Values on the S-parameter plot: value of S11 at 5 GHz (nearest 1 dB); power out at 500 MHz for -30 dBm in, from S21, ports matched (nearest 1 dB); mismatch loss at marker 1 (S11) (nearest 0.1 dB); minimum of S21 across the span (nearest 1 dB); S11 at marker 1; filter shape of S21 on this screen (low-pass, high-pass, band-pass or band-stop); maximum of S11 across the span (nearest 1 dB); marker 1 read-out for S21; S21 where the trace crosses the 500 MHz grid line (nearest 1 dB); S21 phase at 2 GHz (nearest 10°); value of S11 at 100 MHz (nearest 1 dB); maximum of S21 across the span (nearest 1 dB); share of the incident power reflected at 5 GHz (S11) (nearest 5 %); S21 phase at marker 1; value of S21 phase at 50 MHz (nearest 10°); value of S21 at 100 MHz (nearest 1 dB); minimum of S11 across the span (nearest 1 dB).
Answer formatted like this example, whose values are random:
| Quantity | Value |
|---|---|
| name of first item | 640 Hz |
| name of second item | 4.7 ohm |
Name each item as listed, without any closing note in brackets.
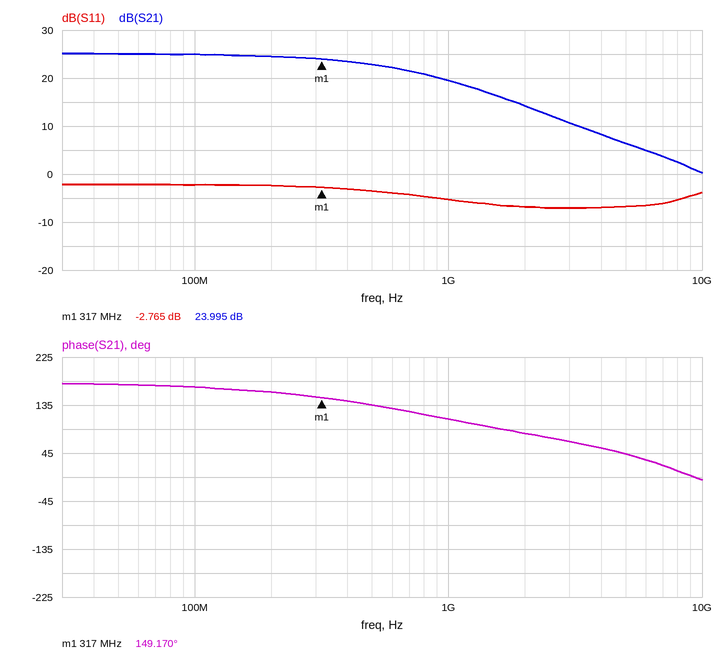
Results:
| Quantity | Value |
|---|---|
| value of S11 at 5 GHz | -7 dB |
| power out at 500 MHz for -30 dBm in, from S21, ports matched | -7 dBm |
| mismatch loss at marker 1 (S11) | 3.3 dB |
| minimum of S21 across the span | 0 dB |
| S11 at marker 1 | -2.765 dB |
| filter shape of S21 on this screen | low-pass |
| maximum of S11 across the span | -2 dB |
| marker 1 read-out for S21 | 23.995 dB |
| S21 where the trace crosses the 500 MHz grid line | 23 dB |
| S21 phase at 2 GHz | 80° |
| value of S11 at 100 MHz | -2 dB |
| maximum of S21 across the span | 25 dB |
| share of the incident power reflected at 5 GHz (S11) | 20 % |
| S21 phase at marker 1 | 149.170° |
| value of S21 phase at 50 MHz | 170° |
| value of S21 at 100 MHz | 25 dB |
| minimum of S11 across the span | -7 dB |
